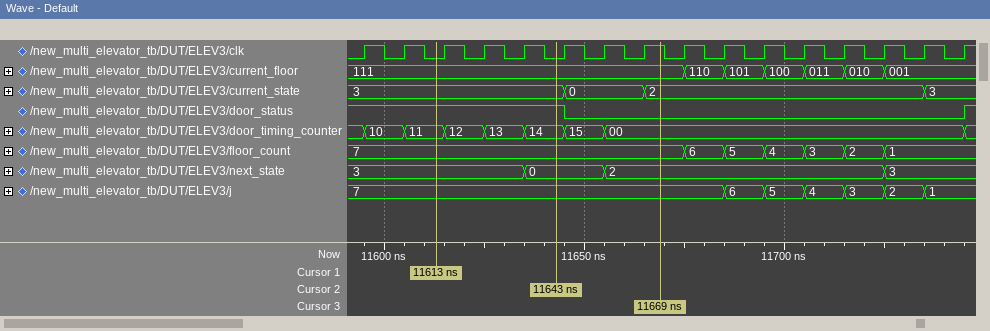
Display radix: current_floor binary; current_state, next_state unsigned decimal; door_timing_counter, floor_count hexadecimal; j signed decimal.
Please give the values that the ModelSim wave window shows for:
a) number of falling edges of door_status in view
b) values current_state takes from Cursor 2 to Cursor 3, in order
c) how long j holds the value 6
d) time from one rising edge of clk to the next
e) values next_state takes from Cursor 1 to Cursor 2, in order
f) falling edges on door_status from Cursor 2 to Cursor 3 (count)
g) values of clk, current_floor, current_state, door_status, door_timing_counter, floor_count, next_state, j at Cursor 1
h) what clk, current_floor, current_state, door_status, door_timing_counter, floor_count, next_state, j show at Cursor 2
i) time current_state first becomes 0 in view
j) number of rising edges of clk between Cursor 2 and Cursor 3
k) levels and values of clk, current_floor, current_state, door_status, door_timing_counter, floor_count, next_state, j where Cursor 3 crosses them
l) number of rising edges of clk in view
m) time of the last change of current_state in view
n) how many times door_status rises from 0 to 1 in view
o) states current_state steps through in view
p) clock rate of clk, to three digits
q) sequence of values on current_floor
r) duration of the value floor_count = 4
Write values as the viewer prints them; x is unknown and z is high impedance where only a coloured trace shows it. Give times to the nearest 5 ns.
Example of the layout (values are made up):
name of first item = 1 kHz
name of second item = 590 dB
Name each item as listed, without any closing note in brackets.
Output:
number of falling edges of door_status in view = 1
values current_state takes from Cursor 2 to Cursor 3, in order = 3, 0, 2
how long j holds the value 6 = 10 ns
time from one rising edge of clk to the next = 10 ns
values next_state takes from Cursor 1 to Cursor 2, in order = 3, 0
falling edges on door_status from Cursor 2 to Cursor 3 = 1
values of clk, current_floor, current_state, door_status, door_timing_counter, floor_count, next_state, j at Cursor 1 = clk=0, current_floor=111, current_state=3, door_status=1, door_timing_counter=11, floor_count=7, next_state=3, j=7
what clk, current_floor, current_state, door_status, door_timing_counter, floor_count, next_state, j show at Cursor 2 = clk=0, current_floor=111, current_state=3, door_status=1, door_timing_counter=14, floor_count=7, next_state=0, j=7
time current_state first becomes 0 in view = 11645 ns
number of rising edges of clk between Cursor 2 and Cursor 3 = 3
levels and values of clk, current_floor, current_state, door_status, door_timing_counter, floor_count, next_state, j where Cursor 3 crosses them = clk=1, current_floor=111, current_state=2, door_status=0, door_timing_counter=00, floor_count=7, next_state=2, j=7
number of rising edges of clk in view = 16
time of the last change of current_state in view = 11735 ns
how many times door_status rises from 0 to 1 in view = 1
states current_state steps through in view = 3, 0, 2, 3
clock rate of clk, to three digits = 100 MHz
sequence of values on current_floor = 111, 110, 101, 100, 011, 010, 001
duration of the value floor_count = 4 = 10 ns
